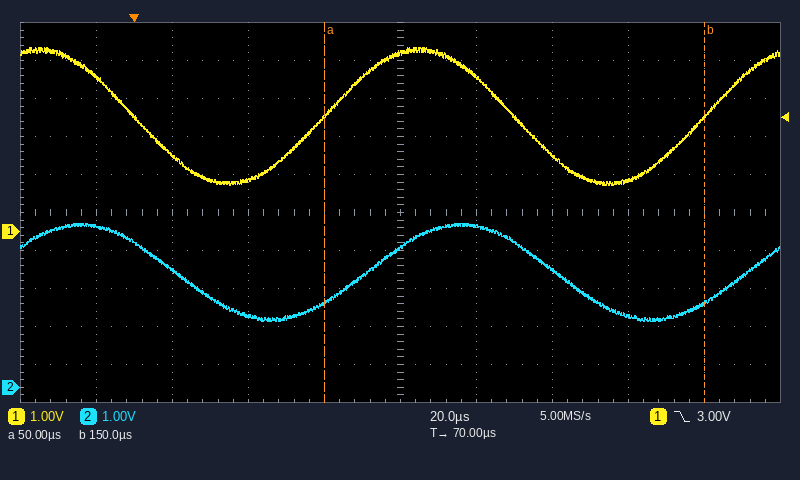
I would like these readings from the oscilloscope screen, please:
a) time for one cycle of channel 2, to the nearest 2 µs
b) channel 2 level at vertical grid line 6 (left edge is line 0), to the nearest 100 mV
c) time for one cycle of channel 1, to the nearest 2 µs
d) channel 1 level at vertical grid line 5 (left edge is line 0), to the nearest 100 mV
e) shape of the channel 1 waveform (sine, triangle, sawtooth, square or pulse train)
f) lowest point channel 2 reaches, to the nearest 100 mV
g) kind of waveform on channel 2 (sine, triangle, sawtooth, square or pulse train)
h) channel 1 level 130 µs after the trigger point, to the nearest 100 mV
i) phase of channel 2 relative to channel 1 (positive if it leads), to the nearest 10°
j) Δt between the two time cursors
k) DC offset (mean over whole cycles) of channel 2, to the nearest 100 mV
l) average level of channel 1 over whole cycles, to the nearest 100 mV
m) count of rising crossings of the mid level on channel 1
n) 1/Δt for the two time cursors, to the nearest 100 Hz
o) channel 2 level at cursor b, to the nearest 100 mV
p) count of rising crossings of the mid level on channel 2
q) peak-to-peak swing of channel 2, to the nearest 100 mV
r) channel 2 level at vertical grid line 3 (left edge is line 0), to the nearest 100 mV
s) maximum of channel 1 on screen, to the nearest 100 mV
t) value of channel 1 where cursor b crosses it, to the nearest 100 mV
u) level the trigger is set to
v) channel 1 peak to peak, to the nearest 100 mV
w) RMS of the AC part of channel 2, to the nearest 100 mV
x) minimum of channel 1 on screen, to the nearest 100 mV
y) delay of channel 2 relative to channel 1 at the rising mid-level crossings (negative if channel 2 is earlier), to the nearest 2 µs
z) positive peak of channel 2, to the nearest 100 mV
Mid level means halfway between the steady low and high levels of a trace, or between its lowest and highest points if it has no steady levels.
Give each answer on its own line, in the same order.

100 µs
4.2 V
100 µs
4.7 V
sine
1.7 V
sine
1.3 V
-40°
100 µs
3.0 V
3.0 V
2
10.0 kHz
2.2 V
2
2.6 V
1.9 V
4.8 V
3.0 V
3.00 V
3.6 V
900 mV
1.2 V
+12 µs
4.3 V
